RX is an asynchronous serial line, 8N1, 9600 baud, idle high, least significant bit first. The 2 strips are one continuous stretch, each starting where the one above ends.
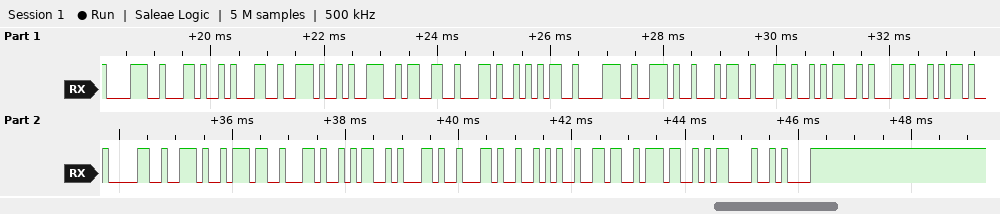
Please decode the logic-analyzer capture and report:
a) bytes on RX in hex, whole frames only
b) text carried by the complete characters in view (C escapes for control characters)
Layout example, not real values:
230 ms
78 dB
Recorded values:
38 2C 31 2E 39 33 2C 35 38 2E 34 2C 4D 2C 2D 30 2E 37 2C 4D 2C 2C 2A 36 37 0D 0A
"8,1.93,58.4,M,-0.7,M,,*67\r\n"
